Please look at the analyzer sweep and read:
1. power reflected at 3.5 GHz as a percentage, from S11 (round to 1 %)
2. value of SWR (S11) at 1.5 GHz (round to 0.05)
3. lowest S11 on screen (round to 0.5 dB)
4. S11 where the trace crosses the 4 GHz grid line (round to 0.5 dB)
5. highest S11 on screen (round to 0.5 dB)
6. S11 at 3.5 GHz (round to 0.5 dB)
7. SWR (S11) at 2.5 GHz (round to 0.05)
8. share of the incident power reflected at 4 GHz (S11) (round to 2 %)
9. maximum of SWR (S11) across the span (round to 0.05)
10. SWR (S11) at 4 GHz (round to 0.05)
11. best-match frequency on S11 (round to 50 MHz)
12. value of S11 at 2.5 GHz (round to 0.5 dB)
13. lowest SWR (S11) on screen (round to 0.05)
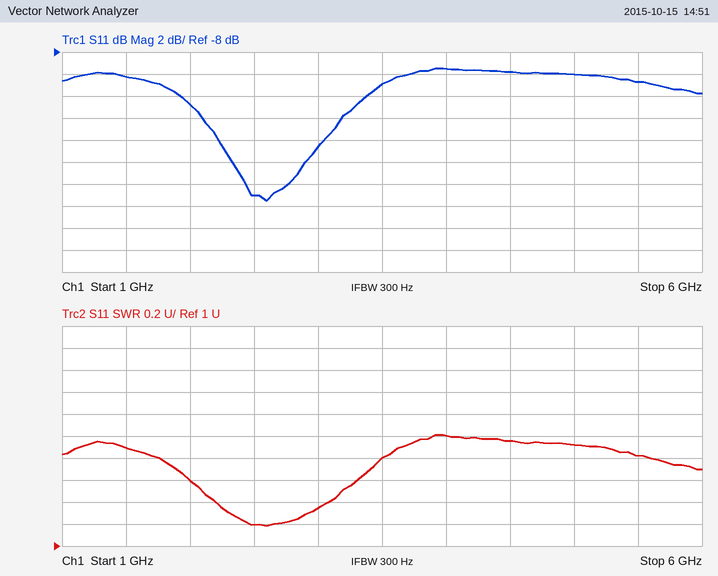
8 %
1.90
-21.5 dB
-9.5 dB
-9.5 dB
-11.0 dB
1.20
12 %
2.00
2.00
2.60 GHz
-21.0 dB
1.20
